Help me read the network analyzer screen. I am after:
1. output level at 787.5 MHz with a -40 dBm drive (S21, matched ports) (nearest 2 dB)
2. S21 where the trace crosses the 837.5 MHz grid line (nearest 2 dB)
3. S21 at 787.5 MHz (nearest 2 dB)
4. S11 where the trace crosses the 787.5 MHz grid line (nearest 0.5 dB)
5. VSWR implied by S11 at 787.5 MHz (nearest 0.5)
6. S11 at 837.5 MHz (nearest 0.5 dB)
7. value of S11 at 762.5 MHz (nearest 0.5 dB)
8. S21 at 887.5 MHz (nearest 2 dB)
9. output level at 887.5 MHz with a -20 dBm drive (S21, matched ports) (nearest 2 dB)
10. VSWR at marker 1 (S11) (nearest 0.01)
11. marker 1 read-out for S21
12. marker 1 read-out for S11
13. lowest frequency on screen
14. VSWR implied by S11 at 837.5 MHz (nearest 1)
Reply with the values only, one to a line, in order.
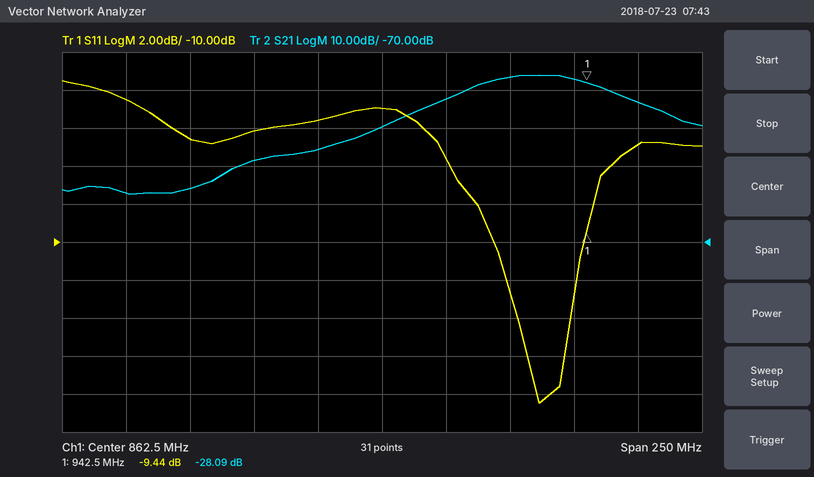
-96 dBm
-46 dB
-56 dB
-4.5 dB
4.0
-3.5 dB
-2.5 dB
-32 dB
-52 dBm
2.02
-28.09 dB
-9.44 dB
737.5 MHz
5
